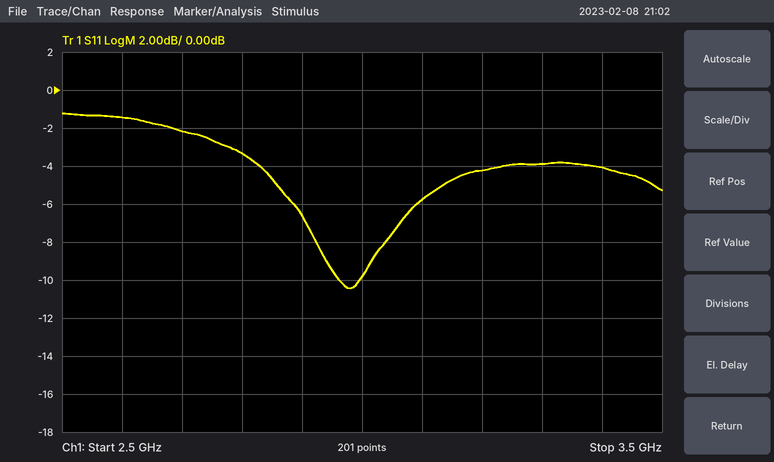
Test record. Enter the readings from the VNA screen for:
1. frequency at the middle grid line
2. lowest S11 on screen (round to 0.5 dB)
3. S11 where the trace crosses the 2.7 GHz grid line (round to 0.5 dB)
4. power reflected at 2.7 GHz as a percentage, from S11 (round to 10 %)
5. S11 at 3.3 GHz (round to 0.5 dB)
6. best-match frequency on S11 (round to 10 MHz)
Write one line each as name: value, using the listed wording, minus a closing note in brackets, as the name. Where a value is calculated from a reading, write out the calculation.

frequency at the middle grid line: 3 GHz
lowest S11 on screen: -10.5 dB
S11 where the trace crosses the 2.7 GHz grid line: -2.0 dB
power reflected at 2.7 GHz as a percentage, from S11: 10^(-2/10) ≈ 63.1 %, so 60 % to the nearest 10 %
S11 at 3.3 GHz: -4.0 dB
best-match frequency on S11: 2.98 GHz
